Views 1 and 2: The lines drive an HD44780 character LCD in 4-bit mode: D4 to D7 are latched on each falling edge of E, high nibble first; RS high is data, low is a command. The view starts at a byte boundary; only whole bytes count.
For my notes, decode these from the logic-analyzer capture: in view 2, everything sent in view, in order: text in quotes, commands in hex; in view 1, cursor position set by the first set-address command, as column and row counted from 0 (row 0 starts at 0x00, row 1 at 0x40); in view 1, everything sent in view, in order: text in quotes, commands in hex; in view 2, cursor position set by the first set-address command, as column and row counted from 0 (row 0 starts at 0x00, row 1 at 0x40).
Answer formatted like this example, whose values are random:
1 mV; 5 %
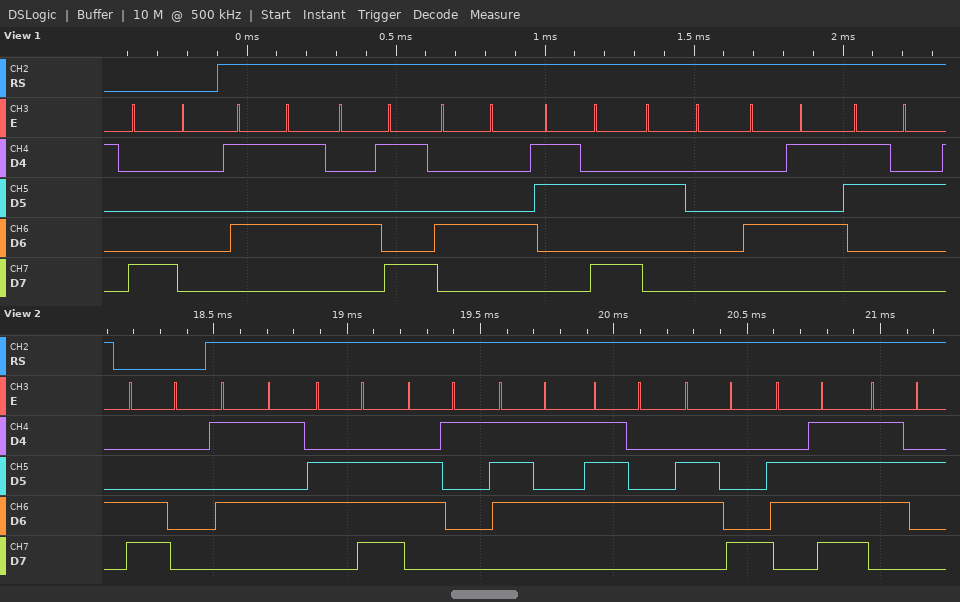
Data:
0xC0 "Unauthor"; column 0, row 0; 0x80 "UID: E2"; column 0, row 1
